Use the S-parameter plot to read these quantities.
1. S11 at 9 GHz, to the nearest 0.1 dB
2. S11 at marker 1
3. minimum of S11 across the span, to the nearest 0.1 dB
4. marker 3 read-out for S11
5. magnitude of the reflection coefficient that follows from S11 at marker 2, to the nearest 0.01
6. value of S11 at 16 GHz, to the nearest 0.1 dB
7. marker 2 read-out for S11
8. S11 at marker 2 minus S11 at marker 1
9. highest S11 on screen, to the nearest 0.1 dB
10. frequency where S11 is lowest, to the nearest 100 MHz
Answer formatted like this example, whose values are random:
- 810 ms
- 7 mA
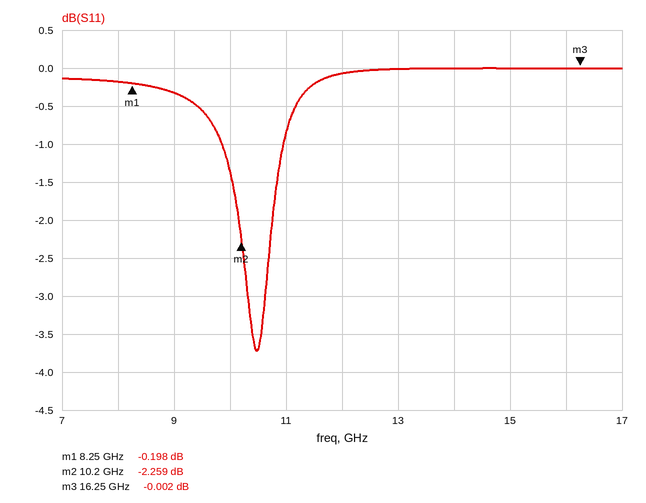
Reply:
- -0.3 dB
- -0.198 dB
- -3.7 dB
- -0.002 dB
- 0.77
- 0.0 dB
- -2.259 dB
- -2.061 dB
- 0.0 dB
- 10.5 GHz
